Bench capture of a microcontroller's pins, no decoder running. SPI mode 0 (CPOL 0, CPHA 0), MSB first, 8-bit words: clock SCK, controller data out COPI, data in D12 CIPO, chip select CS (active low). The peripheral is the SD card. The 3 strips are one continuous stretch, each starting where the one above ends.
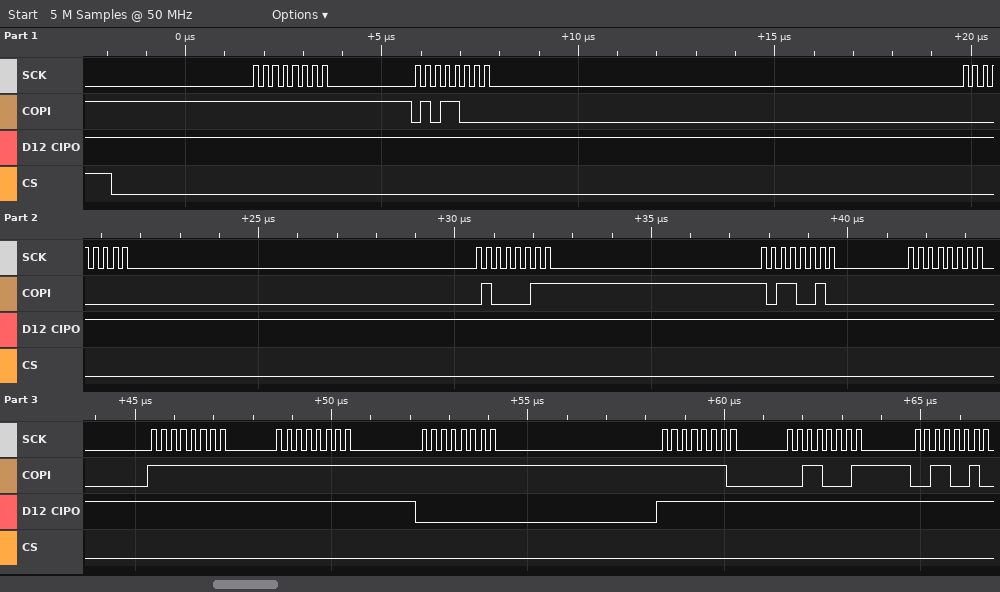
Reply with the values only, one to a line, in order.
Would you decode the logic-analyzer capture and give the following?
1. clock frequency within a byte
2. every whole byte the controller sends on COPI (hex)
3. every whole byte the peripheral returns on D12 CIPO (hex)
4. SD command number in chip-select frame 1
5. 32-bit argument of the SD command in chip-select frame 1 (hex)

4 MHz
FF 58 00 43 B2 00 FF FF FF FE 31 32
FF FF FF FF FF FF FF FF 00 FF FF FF
CMD24
0x0043B200
